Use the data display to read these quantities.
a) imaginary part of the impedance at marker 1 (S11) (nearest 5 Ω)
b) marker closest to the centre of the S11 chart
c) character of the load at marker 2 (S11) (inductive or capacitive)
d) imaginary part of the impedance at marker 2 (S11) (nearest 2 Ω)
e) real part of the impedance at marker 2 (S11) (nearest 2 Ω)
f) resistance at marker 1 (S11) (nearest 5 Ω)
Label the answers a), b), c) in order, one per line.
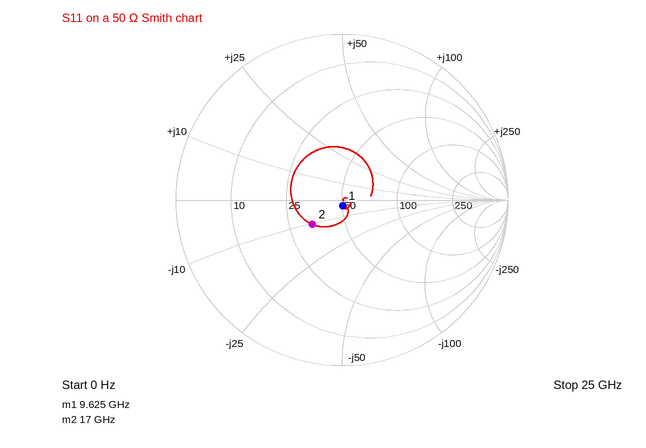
a) -5 Ω
b) marker 1
c) capacitive
d) -10 Ω
e) 34 Ω
f) 50 Ω
